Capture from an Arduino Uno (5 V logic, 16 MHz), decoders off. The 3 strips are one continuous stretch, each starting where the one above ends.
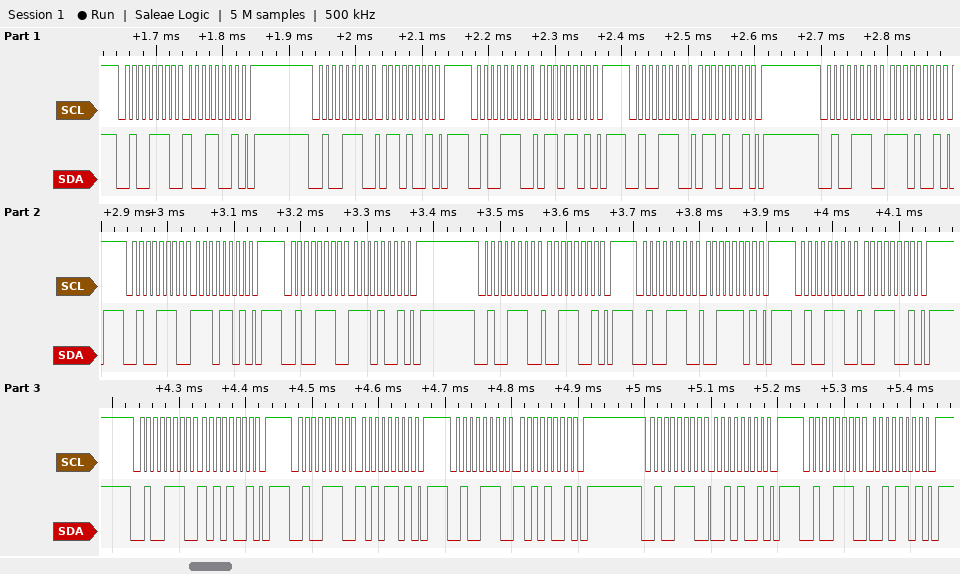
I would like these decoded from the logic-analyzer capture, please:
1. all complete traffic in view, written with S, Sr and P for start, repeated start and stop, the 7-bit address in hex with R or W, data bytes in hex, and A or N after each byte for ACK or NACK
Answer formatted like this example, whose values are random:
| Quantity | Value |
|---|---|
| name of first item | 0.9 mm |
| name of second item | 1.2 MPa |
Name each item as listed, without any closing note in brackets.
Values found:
| Quantity | Value |
|---|---|
| all complete traffic in view, written with S, Sr and P for start, repeated start and stop, the 7-bit address in hex with R or W, data bytes in hex, and A or N after each byte for ACK or NACK | S 27W A 99 A P S 27W A 69 A P S 27W A 6D A P S 27W A 69 A P S 27W A E9 A P S 27W A ED A P S 27W A E9 A P S 27W A 39 A P S 27W A 3D A P S 27W A 39 A P S 27W A A9 A P S 27W A AD A P S 27W A A9 A P S 27W A 29 A P S 27W A 2D A P |
